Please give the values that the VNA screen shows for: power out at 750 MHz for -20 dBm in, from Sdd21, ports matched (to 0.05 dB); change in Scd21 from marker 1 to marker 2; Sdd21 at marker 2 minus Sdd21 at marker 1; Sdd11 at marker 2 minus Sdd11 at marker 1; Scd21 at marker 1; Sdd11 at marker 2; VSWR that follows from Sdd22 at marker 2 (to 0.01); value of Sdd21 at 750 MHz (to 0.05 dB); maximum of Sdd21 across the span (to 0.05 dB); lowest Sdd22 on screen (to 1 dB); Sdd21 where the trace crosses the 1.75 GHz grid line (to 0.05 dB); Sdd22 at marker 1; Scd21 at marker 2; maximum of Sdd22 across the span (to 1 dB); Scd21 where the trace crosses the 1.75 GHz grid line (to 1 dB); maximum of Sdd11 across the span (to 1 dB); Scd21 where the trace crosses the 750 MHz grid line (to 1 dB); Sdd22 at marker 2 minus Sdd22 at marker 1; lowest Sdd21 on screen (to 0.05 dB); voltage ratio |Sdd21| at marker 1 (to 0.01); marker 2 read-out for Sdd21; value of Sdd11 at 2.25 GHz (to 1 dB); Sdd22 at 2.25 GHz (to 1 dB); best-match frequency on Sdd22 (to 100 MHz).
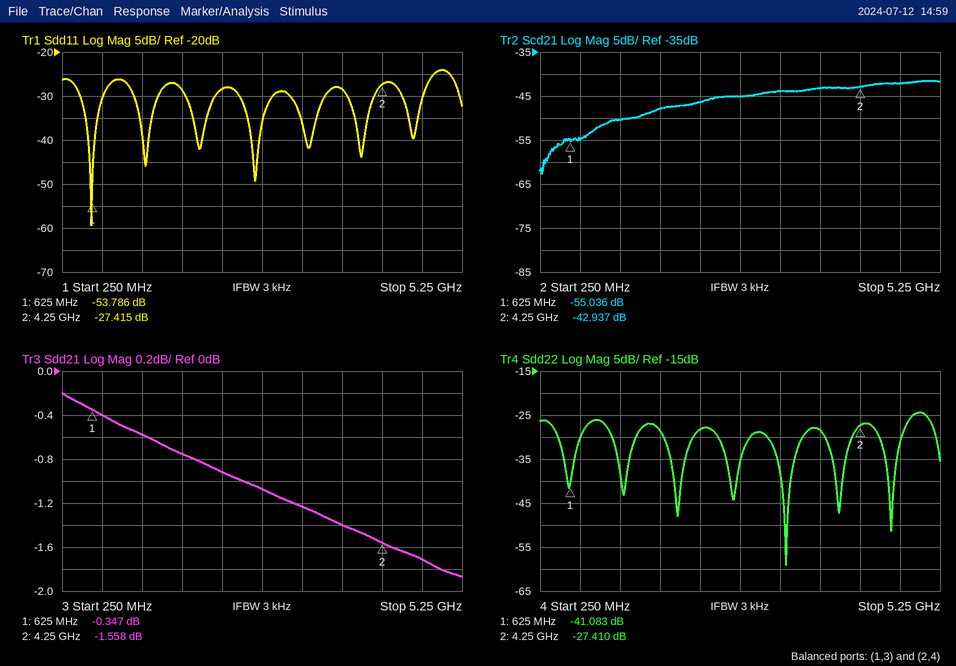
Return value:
-20.40 dBm
12.099 dB
-1.211 dB
26.371 dB
-55.036 dB
-27.415 dB
1.09
-0.40 dB
-0.20 dB
-59 dB
-0.75 dB
-41.083 dB
-42.937 dB
-24 dB
-48 dB
-24 dB
-55 dB
13.673 dB
-1.85 dB
0.96
-1.558 dB
-28 dB
-28 dB
3.3 GHz
